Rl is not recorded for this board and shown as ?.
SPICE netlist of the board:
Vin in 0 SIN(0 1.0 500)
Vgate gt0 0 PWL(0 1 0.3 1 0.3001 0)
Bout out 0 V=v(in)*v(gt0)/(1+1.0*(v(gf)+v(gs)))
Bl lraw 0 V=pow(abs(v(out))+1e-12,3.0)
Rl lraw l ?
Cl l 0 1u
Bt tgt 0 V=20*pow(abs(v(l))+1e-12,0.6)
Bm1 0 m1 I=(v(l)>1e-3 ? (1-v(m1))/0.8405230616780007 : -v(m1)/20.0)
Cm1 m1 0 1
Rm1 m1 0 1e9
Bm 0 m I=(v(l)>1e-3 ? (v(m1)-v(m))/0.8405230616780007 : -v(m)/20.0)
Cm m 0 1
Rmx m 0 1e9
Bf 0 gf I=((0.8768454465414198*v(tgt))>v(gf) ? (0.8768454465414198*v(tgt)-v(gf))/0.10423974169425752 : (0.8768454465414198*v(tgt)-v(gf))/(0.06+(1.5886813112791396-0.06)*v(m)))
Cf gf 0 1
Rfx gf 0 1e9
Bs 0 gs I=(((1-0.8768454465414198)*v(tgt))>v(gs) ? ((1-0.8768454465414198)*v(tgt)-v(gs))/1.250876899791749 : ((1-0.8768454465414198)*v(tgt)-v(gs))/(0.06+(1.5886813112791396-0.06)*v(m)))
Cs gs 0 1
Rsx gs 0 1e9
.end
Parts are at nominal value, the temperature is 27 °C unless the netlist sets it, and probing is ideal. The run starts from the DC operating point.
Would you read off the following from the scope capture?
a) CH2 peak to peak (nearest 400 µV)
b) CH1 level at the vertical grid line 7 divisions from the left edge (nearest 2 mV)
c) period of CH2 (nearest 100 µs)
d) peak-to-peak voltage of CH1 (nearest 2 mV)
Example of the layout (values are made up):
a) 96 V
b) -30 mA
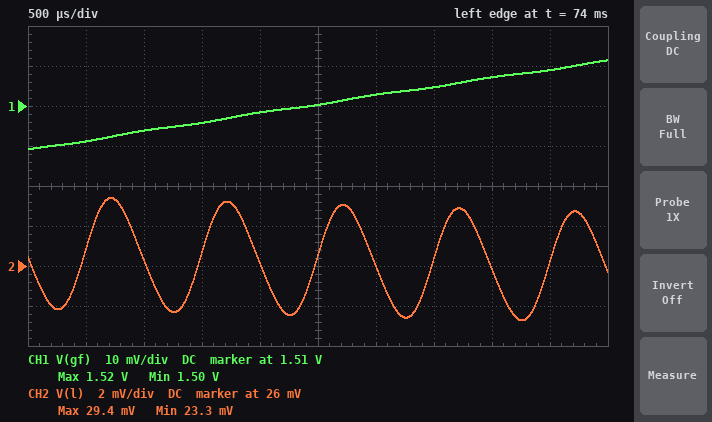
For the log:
a) 6.0 mV
b) 1.514 V
c) 1.0 ms
d) 22 mV
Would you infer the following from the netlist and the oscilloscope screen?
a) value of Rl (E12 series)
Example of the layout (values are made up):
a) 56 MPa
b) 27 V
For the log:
a) 1.8 kΩ
